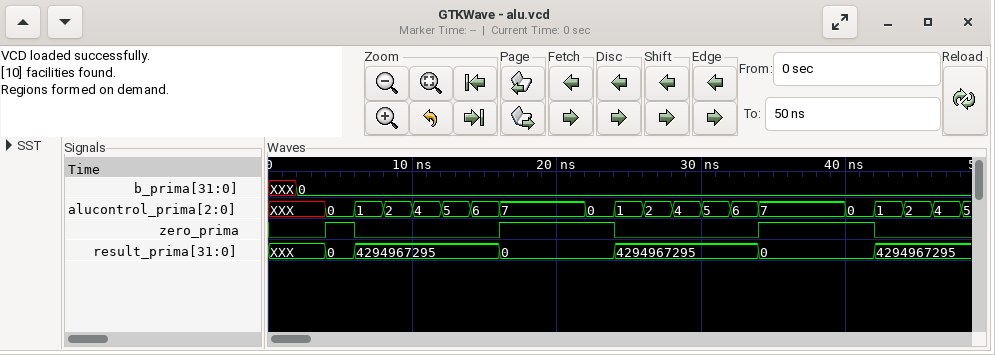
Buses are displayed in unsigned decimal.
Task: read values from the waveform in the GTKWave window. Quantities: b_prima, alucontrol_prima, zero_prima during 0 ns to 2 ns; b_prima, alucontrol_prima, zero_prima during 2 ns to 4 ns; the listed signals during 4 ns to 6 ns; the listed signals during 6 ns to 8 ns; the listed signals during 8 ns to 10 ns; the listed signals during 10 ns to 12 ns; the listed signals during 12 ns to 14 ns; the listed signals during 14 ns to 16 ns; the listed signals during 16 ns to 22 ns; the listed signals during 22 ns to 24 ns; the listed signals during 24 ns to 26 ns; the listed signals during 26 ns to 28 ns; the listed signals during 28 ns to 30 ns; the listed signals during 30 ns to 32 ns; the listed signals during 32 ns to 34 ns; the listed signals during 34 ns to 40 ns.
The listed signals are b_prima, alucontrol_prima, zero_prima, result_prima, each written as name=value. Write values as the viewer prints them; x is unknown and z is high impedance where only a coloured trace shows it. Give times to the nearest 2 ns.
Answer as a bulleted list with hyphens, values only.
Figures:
- b_prima=XXX, alucontrol_prima=XXX, zero_prima=0
- b_prima=0, alucontrol_prima=XXX, zero_prima=0
- b_prima=0, alucontrol_prima=0, zero_prima=1, result_prima=0
- b_prima=0, alucontrol_prima=1, zero_prima=0, result_prima=4294967295
- b_prima=0, alucontrol_prima=2, zero_prima=0, result_prima=4294967295
- b_prima=0, alucontrol_prima=4, zero_prima=0, result_prima=4294967295
- b_prima=0, alucontrol_prima=5, zero_prima=0, result_prima=4294967295
- b_prima=0, alucontrol_prima=6, zero_prima=0, result_prima=4294967295
- b_prima=0, alucontrol_prima=7, zero_prima=1, result_prima=0
- b_prima=0, alucontrol_prima=0, zero_prima=1, result_prima=0
- b_prima=0, alucontrol_prima=1, zero_prima=0, result_prima=4294967295
- b_prima=0, alucontrol_prima=2, zero_prima=0, result_prima=4294967295
- b_prima=0, alucontrol_prima=4, zero_prima=0, result_prima=4294967295
- b_prima=0, alucontrol_prima=5, zero_prima=0, result_prima=4294967295
- b_prima=0, alucontrol_prima=6, zero_prima=0, result_prima=4294967295
- b_prima=0, alucontrol_prima=7, zero_prima=1, result_prima=0
